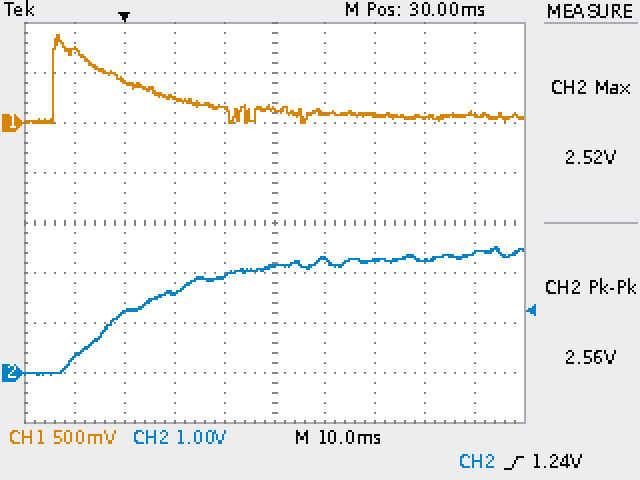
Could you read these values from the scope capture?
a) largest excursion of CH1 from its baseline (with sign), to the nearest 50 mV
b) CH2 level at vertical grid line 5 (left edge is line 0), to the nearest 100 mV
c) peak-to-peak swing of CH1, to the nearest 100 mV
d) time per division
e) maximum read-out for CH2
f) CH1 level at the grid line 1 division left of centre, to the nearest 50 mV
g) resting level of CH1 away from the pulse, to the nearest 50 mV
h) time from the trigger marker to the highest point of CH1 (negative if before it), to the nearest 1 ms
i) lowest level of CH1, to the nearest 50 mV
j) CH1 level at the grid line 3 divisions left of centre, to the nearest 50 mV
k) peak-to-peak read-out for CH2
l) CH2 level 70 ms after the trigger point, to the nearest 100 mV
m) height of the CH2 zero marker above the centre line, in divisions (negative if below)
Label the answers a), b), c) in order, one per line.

a) +800 mV
b) 2.1 V
c) 900 mV
d) 10 ms
e) 2.52 V
f) 150 mV
g) 100 mV
h) -13 ms
i) 0 mV
j) 400 mV
k) 2.56 V
l) 2.4 V
m) -3.0 div
